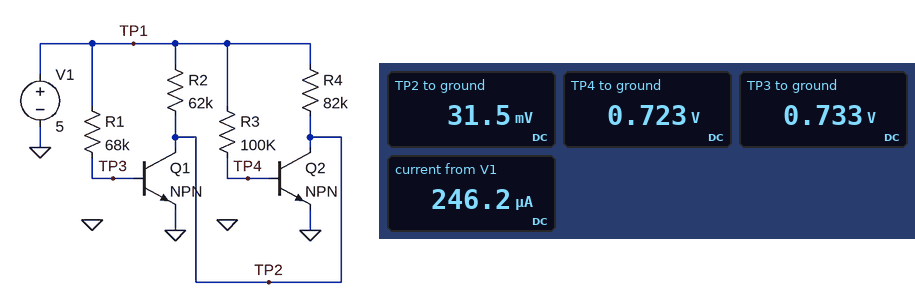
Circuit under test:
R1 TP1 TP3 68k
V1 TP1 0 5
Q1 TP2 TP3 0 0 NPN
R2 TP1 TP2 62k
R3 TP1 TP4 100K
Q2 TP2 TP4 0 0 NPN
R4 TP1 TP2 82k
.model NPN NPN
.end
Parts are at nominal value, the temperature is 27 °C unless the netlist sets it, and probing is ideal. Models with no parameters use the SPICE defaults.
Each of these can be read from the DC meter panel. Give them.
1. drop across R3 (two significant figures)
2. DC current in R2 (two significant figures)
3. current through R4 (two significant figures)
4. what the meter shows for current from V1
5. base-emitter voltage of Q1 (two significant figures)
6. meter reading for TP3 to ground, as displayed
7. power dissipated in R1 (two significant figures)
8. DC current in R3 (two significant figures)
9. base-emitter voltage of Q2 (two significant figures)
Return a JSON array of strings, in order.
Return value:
["4.3 V", "80 µA", "61 µA", "246.2 µA", "730 mV", "0.733 V", "270 µW", "43 µA", "720 mV"]
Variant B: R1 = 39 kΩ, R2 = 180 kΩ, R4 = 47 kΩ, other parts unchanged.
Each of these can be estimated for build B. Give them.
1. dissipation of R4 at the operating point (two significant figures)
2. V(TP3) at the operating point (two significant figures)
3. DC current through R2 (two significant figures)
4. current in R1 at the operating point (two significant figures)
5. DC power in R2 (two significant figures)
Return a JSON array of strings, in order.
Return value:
["530 µW", "740 mV", "28 µA", "110 µA", "140 µW"]
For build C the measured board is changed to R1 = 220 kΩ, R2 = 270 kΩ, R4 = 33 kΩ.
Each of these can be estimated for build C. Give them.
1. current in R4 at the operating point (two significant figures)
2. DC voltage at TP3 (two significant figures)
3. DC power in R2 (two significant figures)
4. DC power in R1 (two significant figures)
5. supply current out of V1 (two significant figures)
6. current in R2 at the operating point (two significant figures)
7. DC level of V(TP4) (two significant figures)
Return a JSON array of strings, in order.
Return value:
["150 µA", "710 mV", "91 µW", "84 µW", "230 µA", "18 µA", "730 mV"]
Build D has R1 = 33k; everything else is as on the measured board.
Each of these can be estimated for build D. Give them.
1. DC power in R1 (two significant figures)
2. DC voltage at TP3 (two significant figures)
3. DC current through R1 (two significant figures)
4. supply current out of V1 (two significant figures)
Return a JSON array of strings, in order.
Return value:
["550 µW", "750 mV", "130 µA", "310 µA"]
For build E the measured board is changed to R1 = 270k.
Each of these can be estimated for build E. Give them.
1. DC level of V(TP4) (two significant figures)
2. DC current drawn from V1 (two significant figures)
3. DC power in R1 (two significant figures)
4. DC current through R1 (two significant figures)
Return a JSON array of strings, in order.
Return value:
["730 mV", "200 µA", "68 µW", "16 µA"]
